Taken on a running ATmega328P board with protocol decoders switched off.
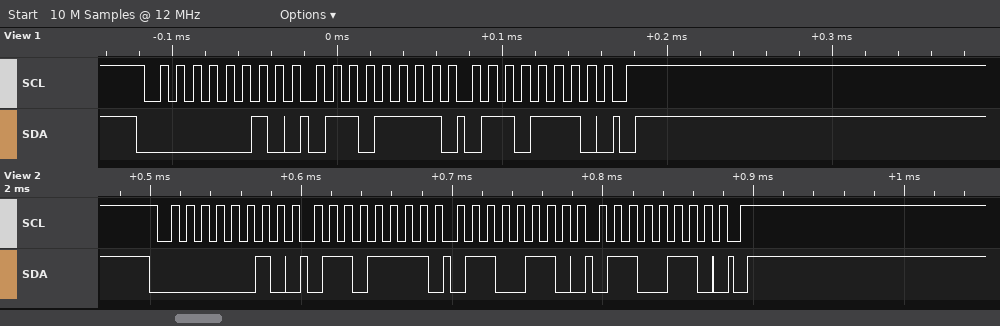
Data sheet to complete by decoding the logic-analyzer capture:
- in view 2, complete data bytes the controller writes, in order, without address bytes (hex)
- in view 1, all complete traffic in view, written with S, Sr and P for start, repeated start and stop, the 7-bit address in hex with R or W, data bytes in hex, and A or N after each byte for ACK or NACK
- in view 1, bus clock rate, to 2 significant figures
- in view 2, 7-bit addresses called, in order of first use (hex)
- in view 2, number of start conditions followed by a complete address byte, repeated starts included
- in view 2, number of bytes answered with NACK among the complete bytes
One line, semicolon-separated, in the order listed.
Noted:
6F 66 66; S 01W A 6F A 6E A P; 100 kHz; 0x01; 1; 0
